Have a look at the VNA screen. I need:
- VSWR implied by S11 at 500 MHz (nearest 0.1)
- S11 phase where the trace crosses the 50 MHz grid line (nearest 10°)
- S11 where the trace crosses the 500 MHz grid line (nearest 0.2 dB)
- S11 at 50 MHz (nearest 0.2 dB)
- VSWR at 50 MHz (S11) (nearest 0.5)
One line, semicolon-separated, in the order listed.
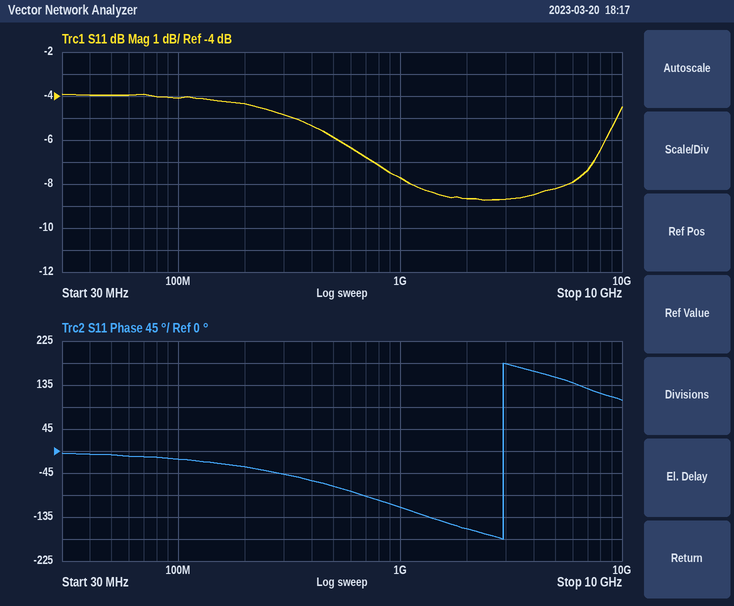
3.1; -10°; -5.8 dB; -4.0 dB; 4.5
